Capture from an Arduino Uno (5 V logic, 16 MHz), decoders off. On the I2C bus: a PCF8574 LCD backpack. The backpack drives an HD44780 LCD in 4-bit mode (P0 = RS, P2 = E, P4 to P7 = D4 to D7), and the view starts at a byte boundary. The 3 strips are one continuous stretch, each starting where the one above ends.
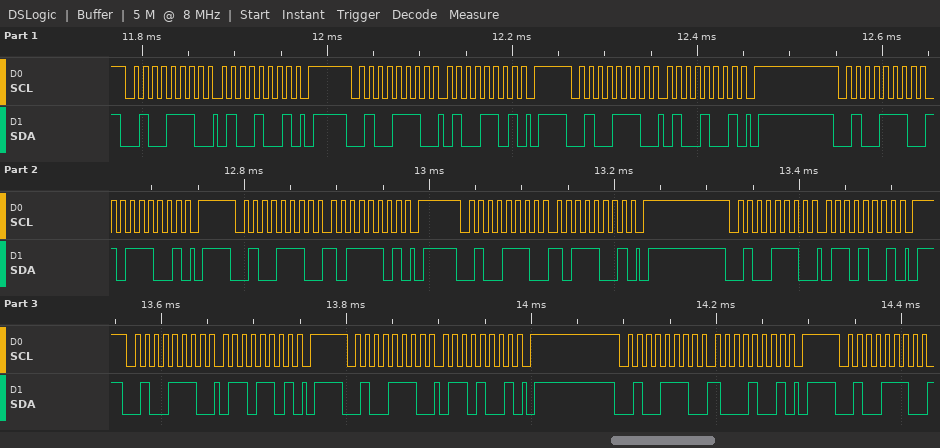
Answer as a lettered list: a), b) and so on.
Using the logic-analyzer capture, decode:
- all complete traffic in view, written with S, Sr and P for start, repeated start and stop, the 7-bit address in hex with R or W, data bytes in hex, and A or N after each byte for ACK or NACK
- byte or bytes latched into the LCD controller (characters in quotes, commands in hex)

a) S 27W A 49 A P S 27W A 4D A P S 27W A 49 A P S 27W A B9 A P S 27W A BD A P S 27W A B9 A P S 27W A 69 A P S 27W A 6D A P S 27W A 69 A P S 27W A 89 A P S 27W A
b) 'K'
